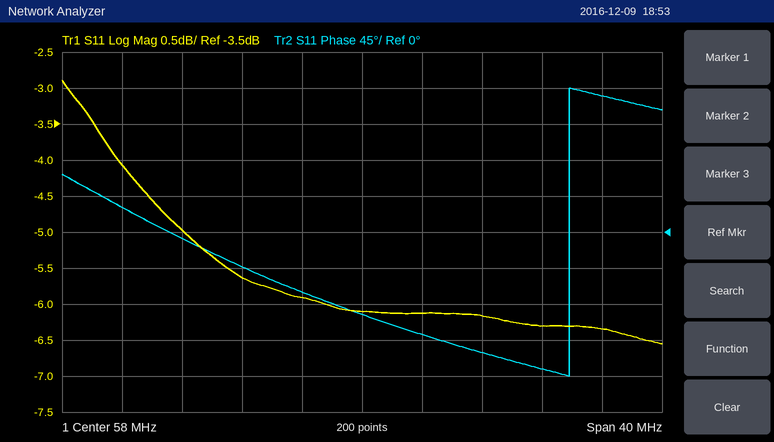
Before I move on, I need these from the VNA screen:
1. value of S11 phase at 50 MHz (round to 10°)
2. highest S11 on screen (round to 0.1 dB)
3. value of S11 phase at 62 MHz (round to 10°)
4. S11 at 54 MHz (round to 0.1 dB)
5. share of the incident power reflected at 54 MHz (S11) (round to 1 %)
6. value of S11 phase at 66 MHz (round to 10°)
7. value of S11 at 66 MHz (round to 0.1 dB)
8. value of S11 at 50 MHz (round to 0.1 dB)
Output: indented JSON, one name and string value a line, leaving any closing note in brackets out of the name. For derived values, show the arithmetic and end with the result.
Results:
{
  "value of S11 phase at 50 MHz": "-40°",
  "highest S11 on screen": "-2.9 dB",
  "value of S11 phase at 62 MHz": "-130°",
  "S11 at 54 MHz": "-5.9 dB",
  "share of the incident power reflected at 54 MHz (S11)": "10^(-5.9/10) ≈ 26 %",
  "value of S11 phase at 66 MHz": "-150°",
  "value of S11 at 66 MHz": "-6.2 dB",
  "value of S11 at 50 MHz": "-5.6 dB"
}
